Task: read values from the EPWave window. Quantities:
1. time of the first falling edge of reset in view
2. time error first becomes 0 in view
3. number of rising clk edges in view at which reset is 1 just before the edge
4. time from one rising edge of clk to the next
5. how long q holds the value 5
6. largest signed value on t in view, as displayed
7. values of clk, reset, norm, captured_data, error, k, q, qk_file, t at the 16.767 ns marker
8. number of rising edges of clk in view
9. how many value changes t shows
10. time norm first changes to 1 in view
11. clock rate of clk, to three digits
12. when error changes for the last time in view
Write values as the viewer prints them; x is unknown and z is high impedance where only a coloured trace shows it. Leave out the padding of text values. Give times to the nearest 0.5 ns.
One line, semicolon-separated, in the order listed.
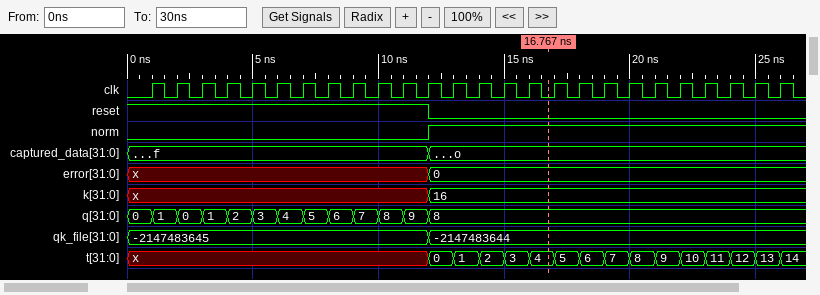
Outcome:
12 ns; 12 ns; 12; 1 ns; 1 ns; 14; clk=0, reset=0, norm=1, captured_data=o, error=0, k=16, q=8, qk_file=-2147483644, t=4; 26; 15; 12 ns; 1.00 GHz; 12 ns
